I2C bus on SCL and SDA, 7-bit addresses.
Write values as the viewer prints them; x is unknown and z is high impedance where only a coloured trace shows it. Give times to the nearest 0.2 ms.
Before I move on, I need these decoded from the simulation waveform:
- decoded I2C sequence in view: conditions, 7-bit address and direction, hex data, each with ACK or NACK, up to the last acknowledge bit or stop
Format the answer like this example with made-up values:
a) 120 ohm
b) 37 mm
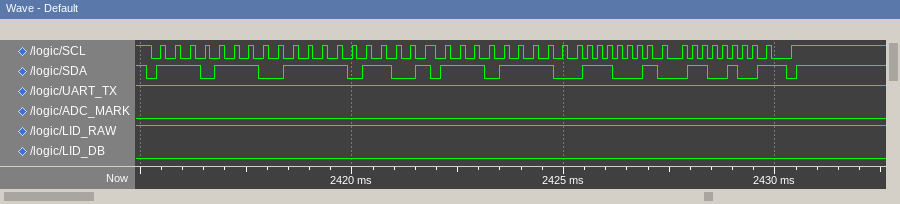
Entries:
a) start, address 77 write ACK, F6 ACK, repeated start, address 77 read ACK, 71 ACK, 64 NACK, stop
